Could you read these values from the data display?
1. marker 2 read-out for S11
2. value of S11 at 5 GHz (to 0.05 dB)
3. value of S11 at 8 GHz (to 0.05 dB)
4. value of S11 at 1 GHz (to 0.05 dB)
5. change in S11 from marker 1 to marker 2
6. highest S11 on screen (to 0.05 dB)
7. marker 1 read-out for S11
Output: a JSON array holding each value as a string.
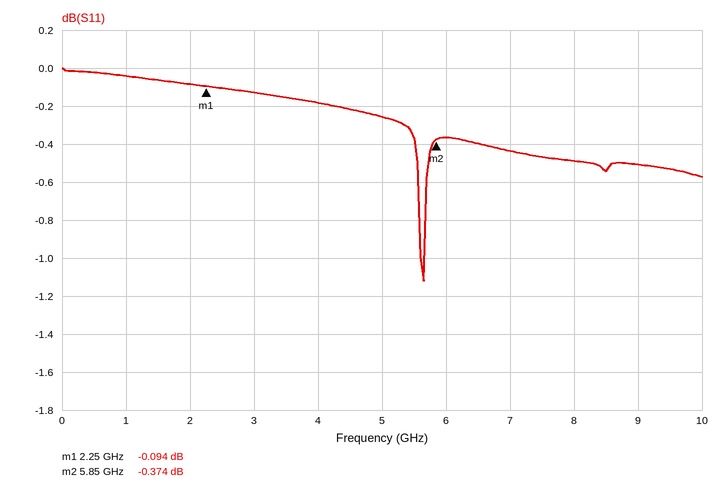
["-0.374 dB", "-0.25 dB", "-0.50 dB", "-0.05 dB", "-0.280 dB", "0.00 dB", "-0.094 dB"]
